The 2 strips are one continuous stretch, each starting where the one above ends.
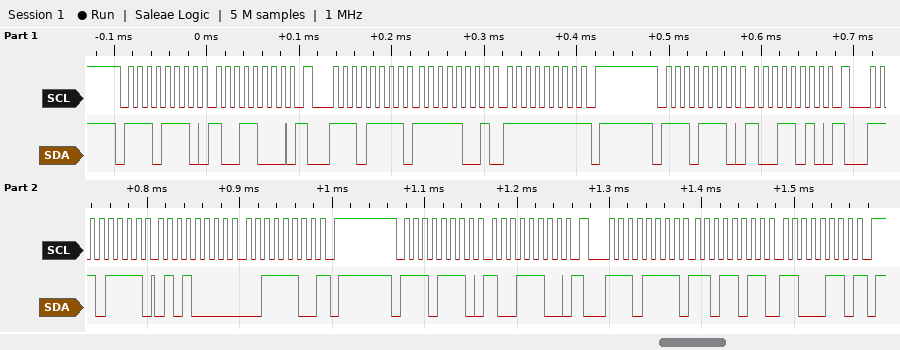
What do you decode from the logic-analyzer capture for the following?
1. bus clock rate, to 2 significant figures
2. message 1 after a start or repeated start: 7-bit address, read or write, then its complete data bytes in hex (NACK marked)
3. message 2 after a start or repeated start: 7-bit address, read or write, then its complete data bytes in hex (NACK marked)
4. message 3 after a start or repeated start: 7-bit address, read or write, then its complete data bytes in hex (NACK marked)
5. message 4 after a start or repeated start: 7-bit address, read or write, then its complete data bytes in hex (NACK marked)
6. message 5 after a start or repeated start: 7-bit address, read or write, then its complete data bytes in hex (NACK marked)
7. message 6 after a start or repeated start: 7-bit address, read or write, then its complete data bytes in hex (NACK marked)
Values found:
100 kHz
0x77 write: 98
0x77 read: F9 FF NACK
0x77 write: 9A
0x77 read: 50 3C NACK
0x77 write: 9C
0x77 read: DB C6 NACK
